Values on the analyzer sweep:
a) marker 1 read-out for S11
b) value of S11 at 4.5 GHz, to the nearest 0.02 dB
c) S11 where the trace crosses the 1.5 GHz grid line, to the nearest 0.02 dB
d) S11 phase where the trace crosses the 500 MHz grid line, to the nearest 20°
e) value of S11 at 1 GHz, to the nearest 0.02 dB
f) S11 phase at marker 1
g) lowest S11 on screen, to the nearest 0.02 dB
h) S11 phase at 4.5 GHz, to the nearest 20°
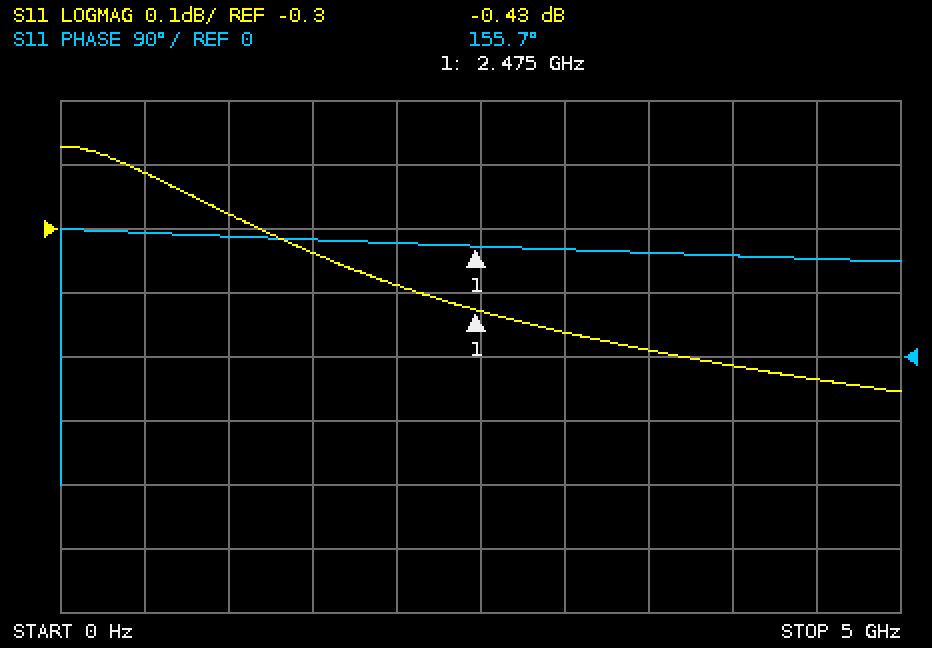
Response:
-0.43 dB
-0.54 dB
-0.34 dB
180°
-0.28 dB
155.7°
-0.56 dB
140°
